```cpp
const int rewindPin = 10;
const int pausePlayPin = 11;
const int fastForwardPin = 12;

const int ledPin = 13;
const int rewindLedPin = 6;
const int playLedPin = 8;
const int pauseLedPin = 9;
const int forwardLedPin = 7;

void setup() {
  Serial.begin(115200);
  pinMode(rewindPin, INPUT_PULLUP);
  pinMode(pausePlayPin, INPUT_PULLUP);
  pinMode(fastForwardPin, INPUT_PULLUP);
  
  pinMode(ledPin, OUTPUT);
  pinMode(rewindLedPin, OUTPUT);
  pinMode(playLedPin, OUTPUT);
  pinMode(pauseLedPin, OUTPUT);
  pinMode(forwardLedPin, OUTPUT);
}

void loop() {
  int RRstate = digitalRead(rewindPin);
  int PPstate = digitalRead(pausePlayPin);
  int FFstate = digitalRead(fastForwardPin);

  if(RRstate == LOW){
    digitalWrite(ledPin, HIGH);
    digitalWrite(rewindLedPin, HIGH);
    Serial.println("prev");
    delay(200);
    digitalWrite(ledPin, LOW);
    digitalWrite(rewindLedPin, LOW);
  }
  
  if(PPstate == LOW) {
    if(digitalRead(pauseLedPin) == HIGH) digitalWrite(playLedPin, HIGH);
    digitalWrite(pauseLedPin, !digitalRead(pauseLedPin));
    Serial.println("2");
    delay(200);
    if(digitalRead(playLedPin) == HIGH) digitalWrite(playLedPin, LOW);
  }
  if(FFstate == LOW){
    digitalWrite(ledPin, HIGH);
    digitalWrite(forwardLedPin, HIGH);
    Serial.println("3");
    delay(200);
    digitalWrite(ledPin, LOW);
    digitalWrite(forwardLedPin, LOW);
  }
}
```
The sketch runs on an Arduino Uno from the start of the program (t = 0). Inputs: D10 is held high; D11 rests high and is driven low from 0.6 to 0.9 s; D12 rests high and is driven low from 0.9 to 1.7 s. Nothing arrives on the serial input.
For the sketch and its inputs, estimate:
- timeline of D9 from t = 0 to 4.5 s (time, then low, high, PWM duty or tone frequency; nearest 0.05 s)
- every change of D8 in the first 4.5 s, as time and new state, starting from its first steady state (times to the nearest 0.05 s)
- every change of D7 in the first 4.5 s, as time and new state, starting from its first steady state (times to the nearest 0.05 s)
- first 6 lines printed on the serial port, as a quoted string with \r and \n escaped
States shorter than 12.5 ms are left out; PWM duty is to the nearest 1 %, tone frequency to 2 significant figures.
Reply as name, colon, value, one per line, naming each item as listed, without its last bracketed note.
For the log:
timeline of D9 from t = 0 to 4.5 s: 0 s low; 0.6 s high; 0.8 s low
every change of D8 in the first 4.5 s, as time and new state, starting from its first steady state: 0 s low; 0.8 s high; 1 s low
every change of D7 in the first 4.5 s, as time and new state, starting from its first steady state: 0 s low; 1 s high; 1.8 s low
first 6 lines printed on the serial port, as a quoted string with \r and \n escaped: "2\r\n2\r\n3\r\n3\r\n3\r\n3\r\n"
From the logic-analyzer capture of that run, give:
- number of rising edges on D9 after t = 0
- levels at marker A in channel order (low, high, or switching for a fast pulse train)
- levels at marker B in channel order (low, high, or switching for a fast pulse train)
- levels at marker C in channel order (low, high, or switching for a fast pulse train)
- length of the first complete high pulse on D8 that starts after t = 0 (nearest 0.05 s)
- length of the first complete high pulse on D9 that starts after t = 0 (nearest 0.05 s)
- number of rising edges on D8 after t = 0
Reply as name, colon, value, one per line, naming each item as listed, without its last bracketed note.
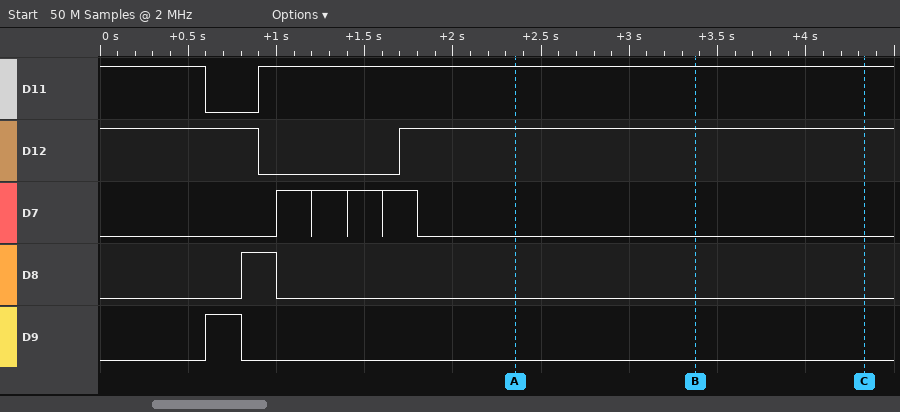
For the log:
number of rising edges on D9 after t = 0: 1
levels at marker A in channel order: D11 high, D12 high, D7 low, D8 low, D9 low
levels at marker B in channel order: D11 high, D12 high, D7 low, D8 low, D9 low
levels at marker C in channel order: D11 high, D12 high, D7 low, D8 low, D9 low
length of the first complete high pulse on D8 that starts after t = 0: 0.20 s
length of the first complete high pulse on D9 that starts after t = 0: 0.20 s
number of rising edges on D8 after t = 0: 1
